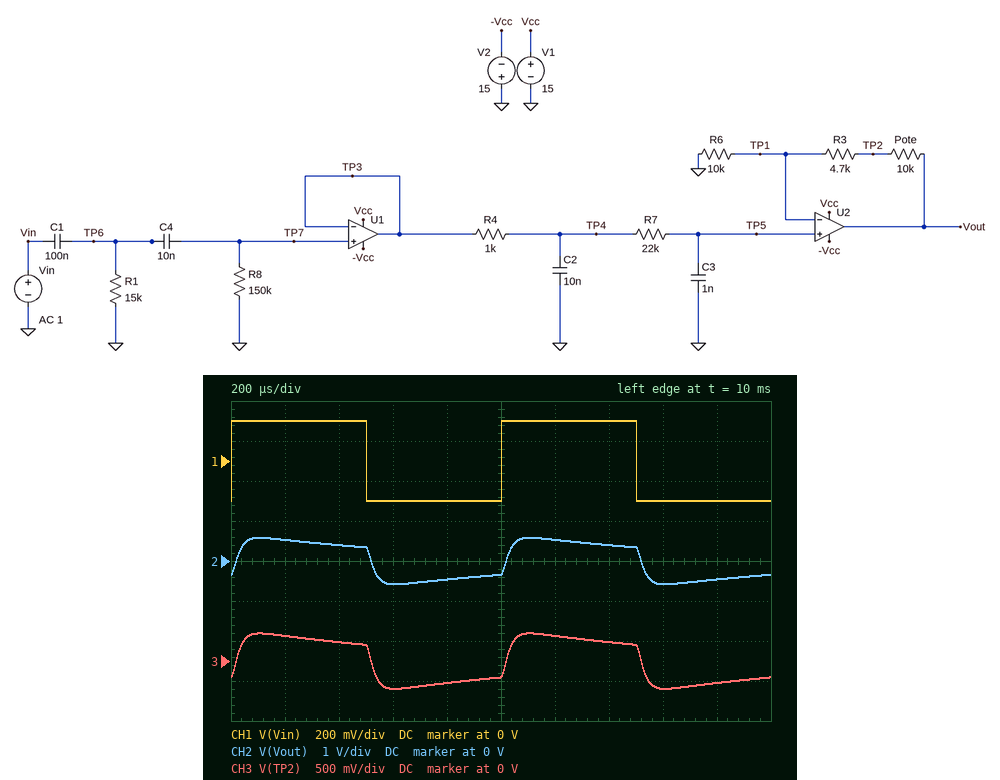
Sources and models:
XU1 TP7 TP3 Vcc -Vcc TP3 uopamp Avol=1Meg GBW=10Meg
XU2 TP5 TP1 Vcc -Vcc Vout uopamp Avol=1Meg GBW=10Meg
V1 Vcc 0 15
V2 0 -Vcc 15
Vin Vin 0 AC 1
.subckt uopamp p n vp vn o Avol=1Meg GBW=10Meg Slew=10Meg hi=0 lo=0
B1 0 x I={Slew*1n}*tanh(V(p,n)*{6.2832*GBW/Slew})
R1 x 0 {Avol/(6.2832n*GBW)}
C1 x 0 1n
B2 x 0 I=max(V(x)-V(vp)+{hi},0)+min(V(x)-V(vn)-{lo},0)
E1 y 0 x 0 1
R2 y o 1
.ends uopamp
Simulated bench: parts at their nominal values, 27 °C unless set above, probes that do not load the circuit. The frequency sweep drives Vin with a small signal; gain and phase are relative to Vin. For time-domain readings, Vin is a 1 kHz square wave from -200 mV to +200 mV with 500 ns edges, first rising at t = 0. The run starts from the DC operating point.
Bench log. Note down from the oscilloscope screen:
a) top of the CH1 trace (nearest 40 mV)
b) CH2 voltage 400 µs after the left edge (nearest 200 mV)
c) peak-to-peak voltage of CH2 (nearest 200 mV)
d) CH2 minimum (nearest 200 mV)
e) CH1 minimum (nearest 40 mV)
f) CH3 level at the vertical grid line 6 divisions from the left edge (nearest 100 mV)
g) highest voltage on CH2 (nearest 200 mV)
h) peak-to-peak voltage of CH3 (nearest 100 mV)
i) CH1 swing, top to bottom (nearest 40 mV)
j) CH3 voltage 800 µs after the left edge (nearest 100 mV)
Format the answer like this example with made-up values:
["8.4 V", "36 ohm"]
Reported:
["200 mV", "400 mV", "1.2 V", "-600 mV", "-200 mV", "300 mV", "600 mV", "700 mV", "400 mV", "-300 mV"]
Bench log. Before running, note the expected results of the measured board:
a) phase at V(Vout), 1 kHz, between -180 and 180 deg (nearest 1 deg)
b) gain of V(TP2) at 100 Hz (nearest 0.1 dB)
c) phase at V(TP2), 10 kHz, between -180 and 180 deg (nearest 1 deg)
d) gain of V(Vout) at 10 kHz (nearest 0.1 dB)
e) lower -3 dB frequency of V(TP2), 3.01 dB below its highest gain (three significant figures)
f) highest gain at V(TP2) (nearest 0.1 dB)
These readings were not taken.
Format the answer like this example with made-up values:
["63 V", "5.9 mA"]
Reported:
["1 deg", "-3.6 dB", "-85 deg", "1.5 dB", "169 Hz", "3.1 dB"]
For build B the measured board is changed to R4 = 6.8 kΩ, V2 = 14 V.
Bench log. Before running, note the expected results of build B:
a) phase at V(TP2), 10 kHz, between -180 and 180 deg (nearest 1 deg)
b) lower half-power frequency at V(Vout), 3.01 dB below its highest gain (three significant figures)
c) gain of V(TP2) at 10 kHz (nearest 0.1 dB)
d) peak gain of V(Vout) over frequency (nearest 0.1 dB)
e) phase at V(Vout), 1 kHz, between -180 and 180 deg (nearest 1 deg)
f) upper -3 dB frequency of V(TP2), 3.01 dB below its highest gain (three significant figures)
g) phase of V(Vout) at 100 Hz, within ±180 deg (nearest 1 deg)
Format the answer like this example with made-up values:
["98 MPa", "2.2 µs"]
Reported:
["-128 deg", "156 Hz", "-14.5 dB", "7.2 dB", "-20 deg", "2.23 kHz", "90 deg"]
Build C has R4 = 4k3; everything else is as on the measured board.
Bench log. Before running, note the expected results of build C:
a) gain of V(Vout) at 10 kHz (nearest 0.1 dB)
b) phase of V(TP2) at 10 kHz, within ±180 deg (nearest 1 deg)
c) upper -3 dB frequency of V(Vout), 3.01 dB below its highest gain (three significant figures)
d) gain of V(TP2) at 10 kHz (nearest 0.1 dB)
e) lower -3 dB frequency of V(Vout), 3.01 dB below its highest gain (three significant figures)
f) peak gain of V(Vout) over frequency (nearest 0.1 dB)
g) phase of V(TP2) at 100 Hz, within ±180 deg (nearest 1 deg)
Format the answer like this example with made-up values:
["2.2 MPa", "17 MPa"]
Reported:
["-6.4 dB", "-121 deg", "3.09 kHz", "-10.9 dB", "162 Hz", "7.4 dB", "91 deg"]
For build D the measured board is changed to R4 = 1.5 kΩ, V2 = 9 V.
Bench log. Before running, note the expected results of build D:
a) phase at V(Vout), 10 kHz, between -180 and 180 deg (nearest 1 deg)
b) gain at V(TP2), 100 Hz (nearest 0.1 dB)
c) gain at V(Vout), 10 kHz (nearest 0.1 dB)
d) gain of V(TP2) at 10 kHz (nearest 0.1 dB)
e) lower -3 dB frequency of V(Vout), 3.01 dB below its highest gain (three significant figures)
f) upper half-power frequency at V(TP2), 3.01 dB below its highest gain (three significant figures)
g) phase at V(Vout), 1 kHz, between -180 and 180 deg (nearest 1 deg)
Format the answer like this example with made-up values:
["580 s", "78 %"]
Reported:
["-96 deg", "-3.6 dB", "0.1 dB", "-4.4 dB", "168 Hz", "5.46 kHz", "-1 deg"]
